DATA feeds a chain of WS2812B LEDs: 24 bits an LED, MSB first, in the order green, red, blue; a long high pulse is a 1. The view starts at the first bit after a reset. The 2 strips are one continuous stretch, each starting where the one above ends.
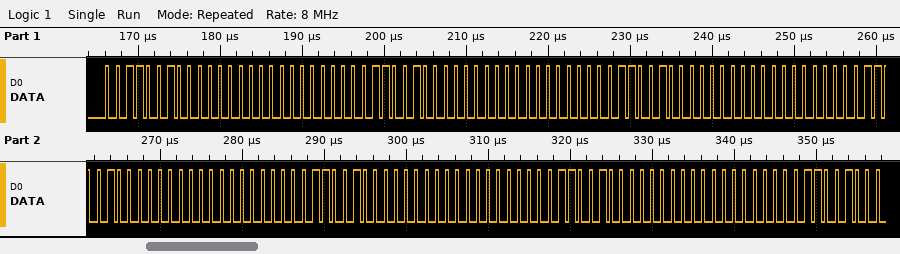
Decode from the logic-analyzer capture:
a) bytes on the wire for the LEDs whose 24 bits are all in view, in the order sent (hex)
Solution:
32 00 00 32 00 00 32 00 00 32 00 00 32 00 00 32 00 00
